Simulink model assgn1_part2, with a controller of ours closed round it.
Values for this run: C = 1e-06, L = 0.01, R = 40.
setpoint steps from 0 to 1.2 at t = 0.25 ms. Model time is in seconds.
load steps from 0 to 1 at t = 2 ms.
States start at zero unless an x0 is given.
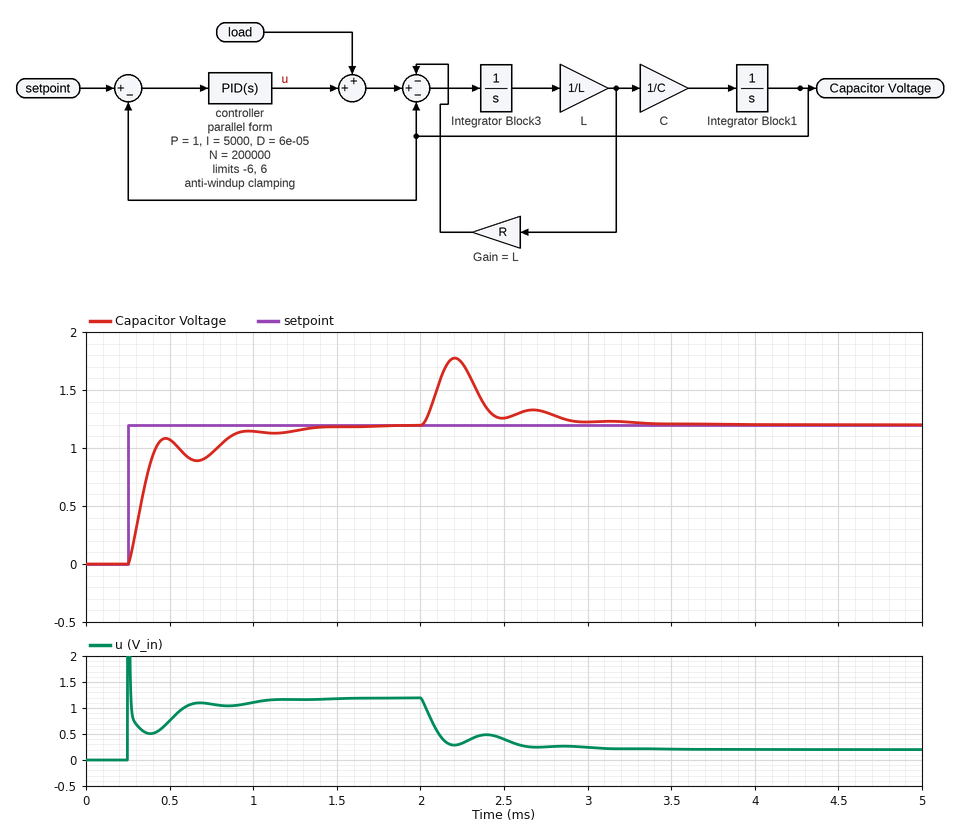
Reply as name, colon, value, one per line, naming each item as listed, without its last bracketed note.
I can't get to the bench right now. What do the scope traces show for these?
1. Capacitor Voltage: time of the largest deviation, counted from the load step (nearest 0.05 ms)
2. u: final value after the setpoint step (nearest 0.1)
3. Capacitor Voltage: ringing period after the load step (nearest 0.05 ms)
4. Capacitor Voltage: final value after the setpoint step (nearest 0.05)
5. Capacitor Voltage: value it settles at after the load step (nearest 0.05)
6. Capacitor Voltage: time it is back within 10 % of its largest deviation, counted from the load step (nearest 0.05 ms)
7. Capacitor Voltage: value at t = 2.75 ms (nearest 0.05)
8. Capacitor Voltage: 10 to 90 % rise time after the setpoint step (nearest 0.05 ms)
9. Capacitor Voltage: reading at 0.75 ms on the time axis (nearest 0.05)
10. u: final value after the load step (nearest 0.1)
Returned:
Capacitor Voltage: time of the largest deviation, counted from the load step: 0.20 ms
u: final value after the setpoint step: 1.2
Capacitor Voltage: ringing period after the load step: 0.45 ms
Capacitor Voltage: final value after the setpoint step: 1.20
Capacitor Voltage: value it settles at after the load step: 1.20
Capacitor Voltage: time it is back within 10 % of its largest deviation, counted from the load step: 0.85 ms
Capacitor Voltage: value at t = 2.75 ms: 1.30
Capacitor Voltage: 10 to 90 % rise time after the setpoint step: 0.20 ms
Capacitor Voltage: reading at 0.75 ms on the time axis: 0.95
u: final value after the load step: 0.2
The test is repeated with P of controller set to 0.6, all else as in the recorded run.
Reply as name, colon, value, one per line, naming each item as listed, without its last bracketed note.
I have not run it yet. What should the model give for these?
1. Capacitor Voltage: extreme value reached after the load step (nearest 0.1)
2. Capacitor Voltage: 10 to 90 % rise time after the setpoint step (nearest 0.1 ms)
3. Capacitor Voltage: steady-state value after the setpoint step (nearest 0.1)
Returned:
Capacitor Voltage: extreme value reached after the load step: 1.9
Capacitor Voltage: 10 to 90 % rise time after the setpoint step: 0.6 ms
Capacitor Voltage: steady-state value after the setpoint step: 1.2
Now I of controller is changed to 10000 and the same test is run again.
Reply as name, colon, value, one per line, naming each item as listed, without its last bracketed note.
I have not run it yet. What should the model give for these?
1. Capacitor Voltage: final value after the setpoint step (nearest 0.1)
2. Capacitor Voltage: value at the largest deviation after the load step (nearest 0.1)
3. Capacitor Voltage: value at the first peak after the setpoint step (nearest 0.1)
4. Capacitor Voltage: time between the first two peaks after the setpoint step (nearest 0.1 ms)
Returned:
Capacitor Voltage: final value after the setpoint step: 1.2
Capacitor Voltage: value at the largest deviation after the load step: 1.7
Capacitor Voltage: value at the first peak after the setpoint step: 1.3
Capacitor Voltage: time between the first two peaks after the setpoint step: 0.5 ms
